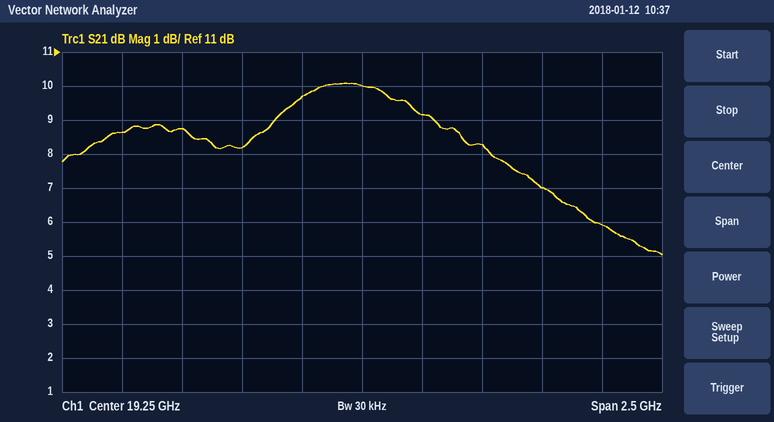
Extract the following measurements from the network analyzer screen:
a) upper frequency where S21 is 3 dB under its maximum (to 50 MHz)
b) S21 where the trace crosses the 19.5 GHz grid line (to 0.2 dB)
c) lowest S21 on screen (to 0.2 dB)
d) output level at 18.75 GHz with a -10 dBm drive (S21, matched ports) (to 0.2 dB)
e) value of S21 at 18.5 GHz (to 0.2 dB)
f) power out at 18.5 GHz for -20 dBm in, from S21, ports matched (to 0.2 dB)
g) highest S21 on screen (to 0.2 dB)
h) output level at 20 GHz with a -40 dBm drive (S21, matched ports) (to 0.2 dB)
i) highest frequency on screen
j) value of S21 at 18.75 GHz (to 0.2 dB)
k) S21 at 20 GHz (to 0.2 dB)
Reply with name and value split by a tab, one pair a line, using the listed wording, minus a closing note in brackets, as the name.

upper frequency where S21 is 3 dB under its maximum	20.00 GHz
S21 where the trace crosses the 19.5 GHz grid line	9.2 dB
lowest S21 on screen	5.0 dB
output level at 18.75 GHz with a -10 dBm drive (S21, matched ports)	-1.8 dBm
value of S21 at 18.5 GHz	8.8 dB
power out at 18.5 GHz for -20 dBm in, from S21, ports matched	-11.2 dBm
highest S21 on screen	10.0 dB
output level at 20 GHz with a -40 dBm drive (S21, matched ports)	-33.0 dBm
highest frequency on screen	20.5 GHz
value of S21 at 18.75 GHz	8.2 dB
S21 at 20 GHz	7.0 dB
